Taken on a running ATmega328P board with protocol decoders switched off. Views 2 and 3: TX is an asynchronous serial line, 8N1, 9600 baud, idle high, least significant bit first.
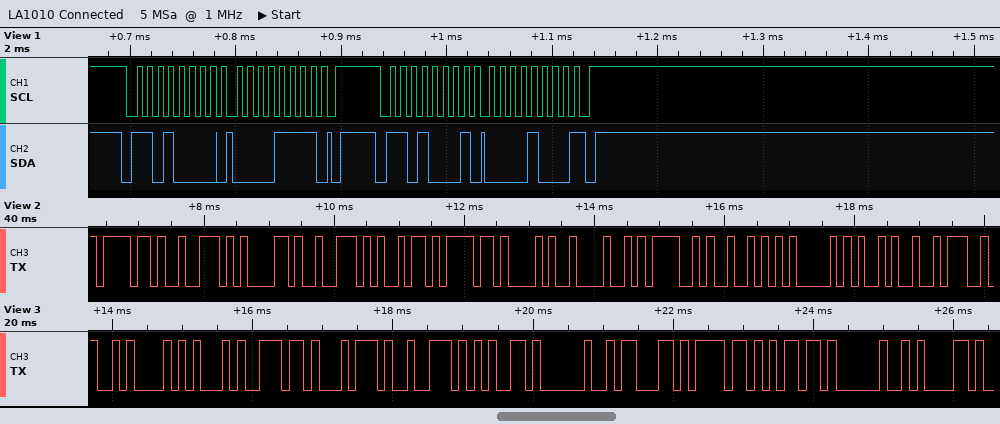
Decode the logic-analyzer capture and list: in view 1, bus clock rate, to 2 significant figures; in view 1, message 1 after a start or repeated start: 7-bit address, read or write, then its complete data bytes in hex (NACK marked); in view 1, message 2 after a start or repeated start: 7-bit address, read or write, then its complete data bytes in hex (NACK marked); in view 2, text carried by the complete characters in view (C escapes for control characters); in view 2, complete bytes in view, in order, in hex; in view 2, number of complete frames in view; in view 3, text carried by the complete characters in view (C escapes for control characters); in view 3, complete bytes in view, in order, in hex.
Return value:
100 kHz
0x68 write: 0F
0x68 read: 08 NACK
"orario(HORA):"
0x6F 0x72 0x61 0x72 0x69 0x6F 0x28 0x48 0x4F 0x52 0x41 0x29 0x3A
13
"\nEntre com a"
0A 45 6E 74 72 65 20 63 6F 6D 20 61
